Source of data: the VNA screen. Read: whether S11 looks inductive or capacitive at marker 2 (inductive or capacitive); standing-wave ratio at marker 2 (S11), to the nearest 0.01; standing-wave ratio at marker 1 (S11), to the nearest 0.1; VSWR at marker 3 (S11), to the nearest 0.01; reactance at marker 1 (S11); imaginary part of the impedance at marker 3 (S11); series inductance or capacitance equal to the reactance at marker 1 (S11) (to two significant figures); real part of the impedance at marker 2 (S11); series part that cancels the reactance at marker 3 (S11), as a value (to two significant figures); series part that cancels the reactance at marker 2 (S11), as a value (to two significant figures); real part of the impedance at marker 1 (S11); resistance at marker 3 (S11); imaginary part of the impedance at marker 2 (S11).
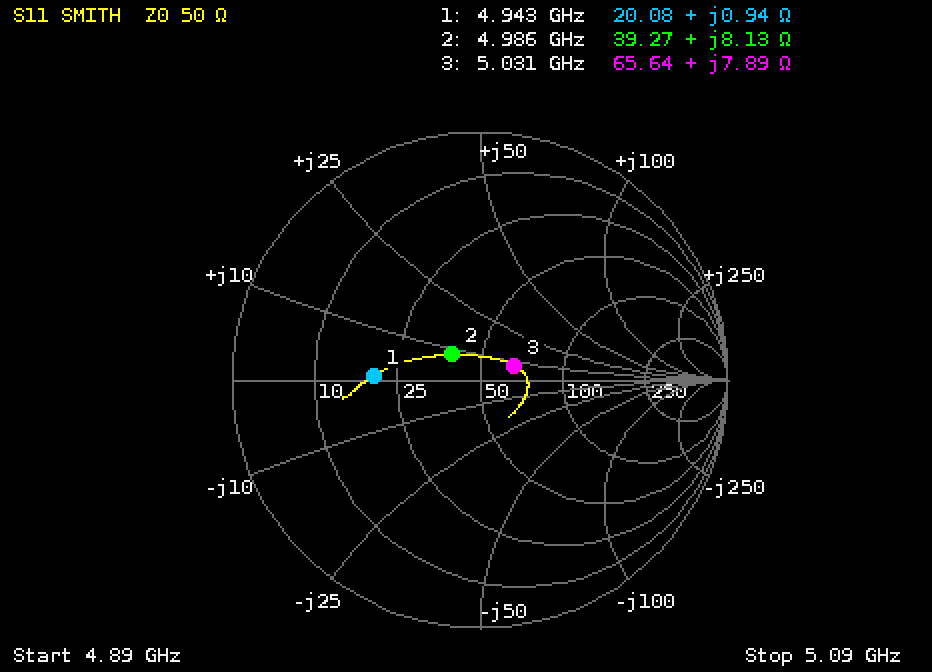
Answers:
inductive
1.35
2.5
1.36
+0.94 Ω
+7.89 Ω
30 pH
39.27 Ω
4.0 pF
3.9 pF
20.08 Ω
65.64 Ω
+8.13 Ω
